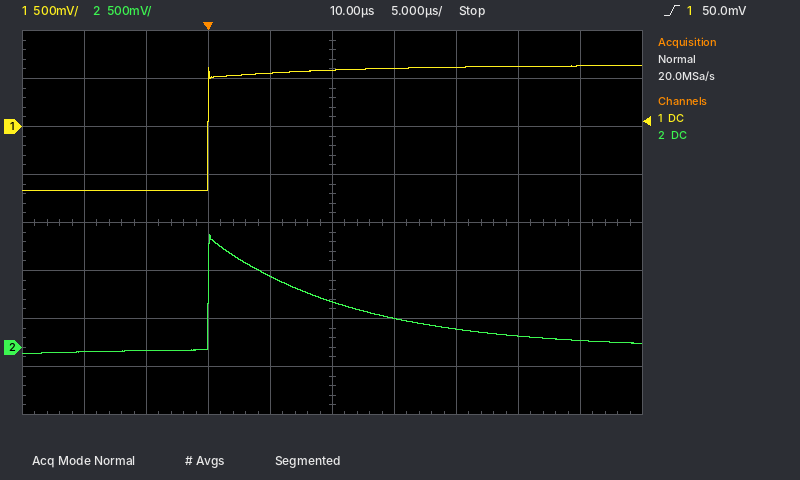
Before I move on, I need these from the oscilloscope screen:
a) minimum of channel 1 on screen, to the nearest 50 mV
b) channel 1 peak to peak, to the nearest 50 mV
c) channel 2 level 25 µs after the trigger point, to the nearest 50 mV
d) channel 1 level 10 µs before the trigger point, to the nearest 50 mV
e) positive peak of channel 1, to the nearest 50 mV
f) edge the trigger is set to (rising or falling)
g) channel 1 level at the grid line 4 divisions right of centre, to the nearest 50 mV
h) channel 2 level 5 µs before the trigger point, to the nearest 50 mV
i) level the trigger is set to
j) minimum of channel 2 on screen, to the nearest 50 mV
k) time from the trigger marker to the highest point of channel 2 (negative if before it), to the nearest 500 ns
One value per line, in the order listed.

-650 mV
1.30 V
100 mV
-650 mV
650 mV
rising
650 mV
-50 mV
50.0 mV
-50 mV
0.0 µs
